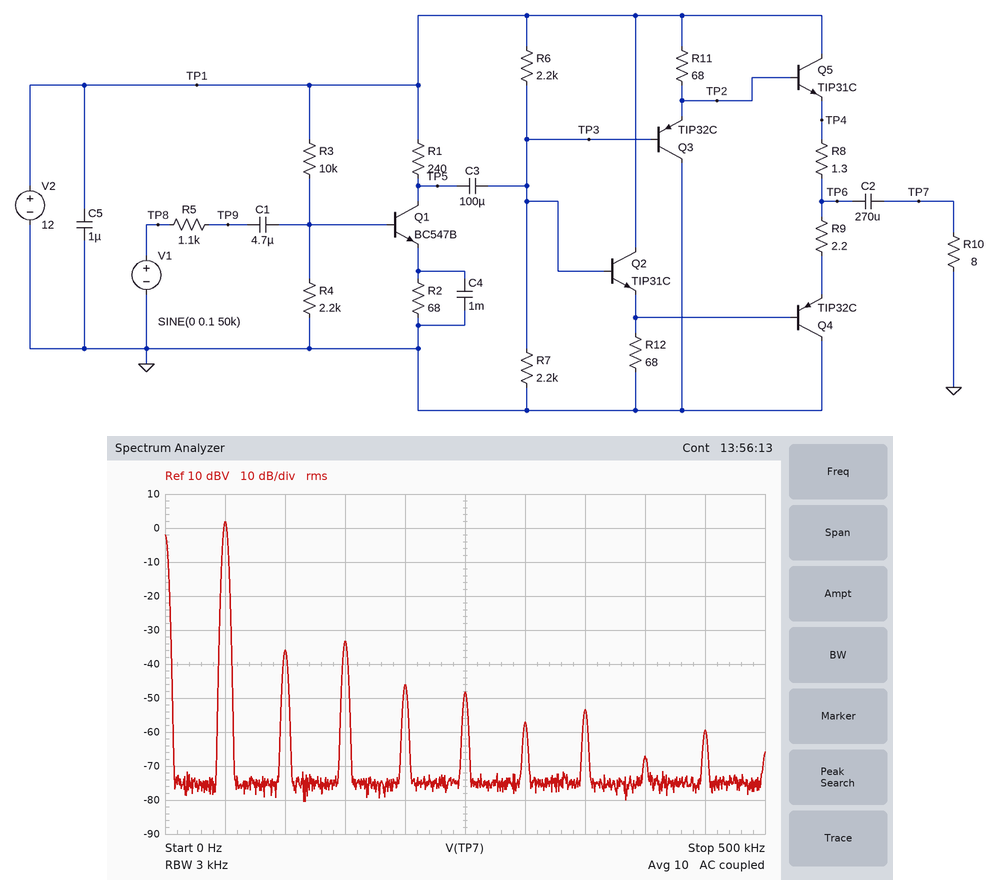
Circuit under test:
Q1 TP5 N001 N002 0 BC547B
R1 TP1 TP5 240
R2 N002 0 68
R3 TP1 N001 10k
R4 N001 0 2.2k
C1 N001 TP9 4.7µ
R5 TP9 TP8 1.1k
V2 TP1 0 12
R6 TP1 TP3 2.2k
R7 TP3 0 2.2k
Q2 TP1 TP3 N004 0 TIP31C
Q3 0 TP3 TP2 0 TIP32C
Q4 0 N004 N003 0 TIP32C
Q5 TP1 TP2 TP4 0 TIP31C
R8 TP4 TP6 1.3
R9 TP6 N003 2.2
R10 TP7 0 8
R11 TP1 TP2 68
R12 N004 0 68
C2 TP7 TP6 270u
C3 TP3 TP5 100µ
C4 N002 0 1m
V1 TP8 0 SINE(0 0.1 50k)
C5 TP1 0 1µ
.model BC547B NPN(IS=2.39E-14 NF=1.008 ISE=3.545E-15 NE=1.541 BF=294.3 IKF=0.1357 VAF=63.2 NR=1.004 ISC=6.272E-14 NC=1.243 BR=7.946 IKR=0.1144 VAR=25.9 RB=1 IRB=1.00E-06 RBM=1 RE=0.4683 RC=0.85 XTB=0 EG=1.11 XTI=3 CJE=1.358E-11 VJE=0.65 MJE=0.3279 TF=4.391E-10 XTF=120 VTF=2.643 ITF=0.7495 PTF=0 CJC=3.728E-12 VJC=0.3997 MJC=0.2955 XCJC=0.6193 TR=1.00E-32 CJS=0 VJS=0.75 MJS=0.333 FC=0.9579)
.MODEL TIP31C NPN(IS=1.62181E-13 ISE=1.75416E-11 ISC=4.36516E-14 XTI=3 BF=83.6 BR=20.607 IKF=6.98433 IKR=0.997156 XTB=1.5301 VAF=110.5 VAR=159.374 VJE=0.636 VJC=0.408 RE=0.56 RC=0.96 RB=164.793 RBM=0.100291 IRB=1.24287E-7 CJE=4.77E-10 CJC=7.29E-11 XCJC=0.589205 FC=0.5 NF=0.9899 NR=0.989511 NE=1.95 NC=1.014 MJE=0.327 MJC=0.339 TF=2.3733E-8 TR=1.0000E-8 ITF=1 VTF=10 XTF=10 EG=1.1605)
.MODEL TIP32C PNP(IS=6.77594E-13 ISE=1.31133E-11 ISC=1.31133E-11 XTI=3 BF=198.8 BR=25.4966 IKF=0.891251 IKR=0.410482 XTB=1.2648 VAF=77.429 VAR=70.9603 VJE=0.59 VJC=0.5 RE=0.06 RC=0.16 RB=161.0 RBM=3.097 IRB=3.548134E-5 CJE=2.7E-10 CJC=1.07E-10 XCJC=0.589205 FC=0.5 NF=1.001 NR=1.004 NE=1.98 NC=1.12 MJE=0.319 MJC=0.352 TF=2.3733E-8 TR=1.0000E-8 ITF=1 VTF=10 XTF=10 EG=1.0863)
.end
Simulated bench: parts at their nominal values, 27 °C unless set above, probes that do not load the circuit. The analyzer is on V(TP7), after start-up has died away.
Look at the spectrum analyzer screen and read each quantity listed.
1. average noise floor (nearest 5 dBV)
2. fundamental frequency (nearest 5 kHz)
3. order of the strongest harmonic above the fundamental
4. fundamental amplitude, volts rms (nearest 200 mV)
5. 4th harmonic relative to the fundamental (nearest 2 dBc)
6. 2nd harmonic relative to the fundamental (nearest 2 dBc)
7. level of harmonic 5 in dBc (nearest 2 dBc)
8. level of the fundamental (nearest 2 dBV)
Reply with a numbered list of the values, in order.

1. -75 dBV
2. 50 kHz
3. 3
4. 1.2 V
5. -48 dBc
6. -38 dBc
7. -50 dBc
8. 2 dBV
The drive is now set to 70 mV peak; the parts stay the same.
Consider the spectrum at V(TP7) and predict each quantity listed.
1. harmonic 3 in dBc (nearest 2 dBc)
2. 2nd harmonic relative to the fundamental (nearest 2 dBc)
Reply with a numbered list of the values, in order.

1. -38 dBc
2. -40 dBc
